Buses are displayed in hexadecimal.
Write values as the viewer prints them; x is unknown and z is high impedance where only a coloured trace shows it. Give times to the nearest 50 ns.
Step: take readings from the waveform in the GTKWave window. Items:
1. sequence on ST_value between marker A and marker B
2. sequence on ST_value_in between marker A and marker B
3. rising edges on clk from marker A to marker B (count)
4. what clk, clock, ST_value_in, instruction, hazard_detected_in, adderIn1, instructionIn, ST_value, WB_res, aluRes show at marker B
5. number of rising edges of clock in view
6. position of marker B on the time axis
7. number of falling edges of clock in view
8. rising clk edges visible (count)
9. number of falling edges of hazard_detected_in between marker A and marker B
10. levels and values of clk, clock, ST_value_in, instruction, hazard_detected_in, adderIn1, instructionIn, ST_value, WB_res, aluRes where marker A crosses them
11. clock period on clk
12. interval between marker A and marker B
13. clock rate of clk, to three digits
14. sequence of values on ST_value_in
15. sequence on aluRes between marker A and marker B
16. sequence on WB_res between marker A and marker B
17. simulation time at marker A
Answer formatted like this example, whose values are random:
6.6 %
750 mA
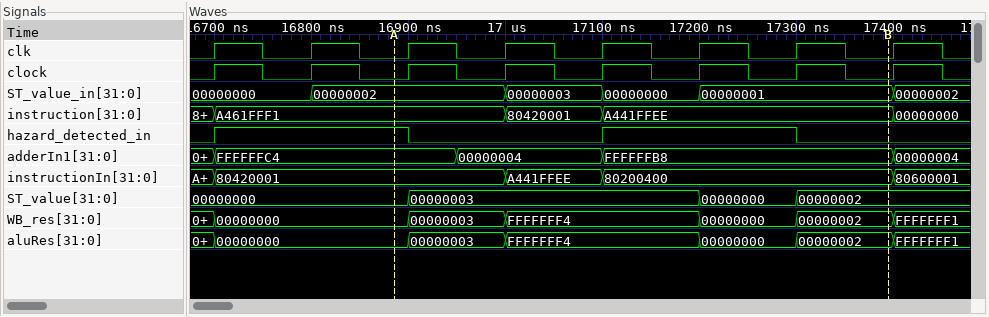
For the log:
00000000, 00000003, 00000000, 00000002
00000002, 00000003, 00000000, 00000001
5
clk=0, clock=0, ST_value_in=00000001, instruction=A441FFEE, hazard_detected_in=0, adderIn1=FFFFFFB8, instructionIn=80200400, ST_value=00000002, WB_res=00000002, aluRes=00000002
8
17400 ns
8
8
2
clk=0, clock=0, ST_value_in=00000002, instruction=A461FFF1, hazard_detected_in=1, adderIn1=FFFFFFC4, instructionIn=80420001, ST_value=00000000, WB_res=00000000, aluRes=00000000
100 ns
500 ns
10.0 MHz
00000000, 00000002, 00000003, 00000000, 00000001, 00000002
00000000, 00000003, FFFFFFF4, 00000000, 00000002
00000000, 00000003, FFFFFFF4, 00000000, 00000002
16900 ns
